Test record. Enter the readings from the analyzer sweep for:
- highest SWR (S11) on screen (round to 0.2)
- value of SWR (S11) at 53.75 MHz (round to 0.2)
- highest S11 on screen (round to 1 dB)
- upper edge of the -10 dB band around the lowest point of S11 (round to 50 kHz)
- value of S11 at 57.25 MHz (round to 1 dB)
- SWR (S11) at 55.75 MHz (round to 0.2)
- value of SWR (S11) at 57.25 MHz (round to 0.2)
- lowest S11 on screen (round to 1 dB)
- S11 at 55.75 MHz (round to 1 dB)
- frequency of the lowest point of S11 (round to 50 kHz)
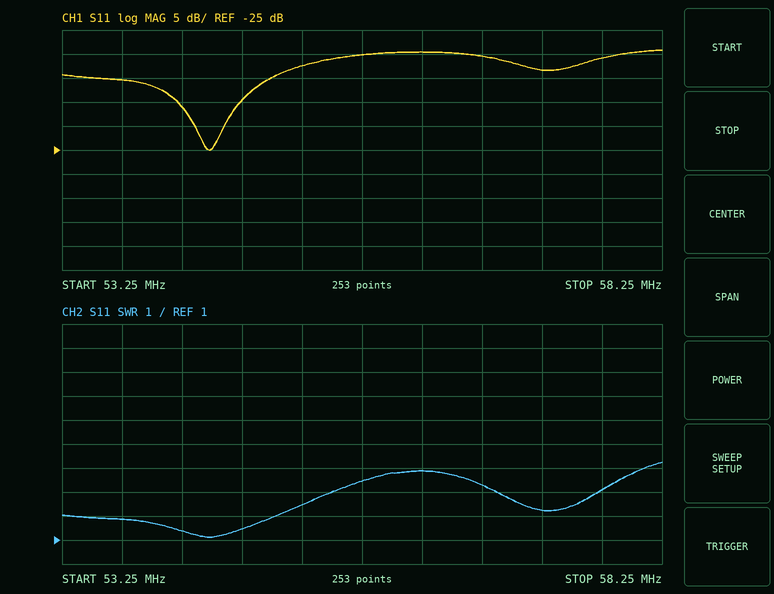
4.2
1.8
-4 dB
55.00 MHz
-8 dB
3.4
2.2
-25 dB
-5 dB
54.50 MHz
